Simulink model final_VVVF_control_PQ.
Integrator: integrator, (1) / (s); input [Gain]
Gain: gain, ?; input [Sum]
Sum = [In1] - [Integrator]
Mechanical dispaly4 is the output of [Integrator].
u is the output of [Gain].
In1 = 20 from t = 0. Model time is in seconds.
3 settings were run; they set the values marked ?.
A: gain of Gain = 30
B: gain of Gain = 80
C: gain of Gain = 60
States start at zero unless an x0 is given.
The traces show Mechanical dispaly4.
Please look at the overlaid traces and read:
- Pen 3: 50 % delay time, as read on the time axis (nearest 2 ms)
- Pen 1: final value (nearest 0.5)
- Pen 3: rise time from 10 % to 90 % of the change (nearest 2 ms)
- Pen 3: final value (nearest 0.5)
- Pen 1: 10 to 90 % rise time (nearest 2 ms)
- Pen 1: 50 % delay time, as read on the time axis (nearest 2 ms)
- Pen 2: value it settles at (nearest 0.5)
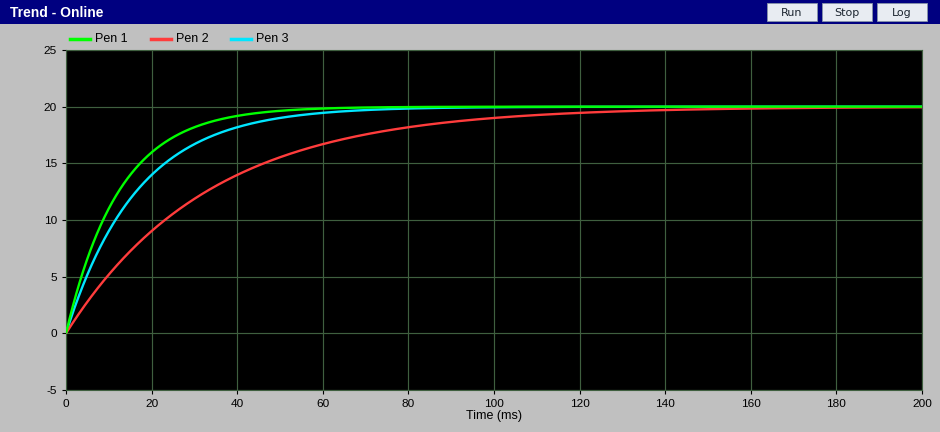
12 ms
20.0
36 ms
20.0
28 ms
8 ms
20.0
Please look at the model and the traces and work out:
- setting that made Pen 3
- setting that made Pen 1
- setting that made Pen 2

C
B
A
